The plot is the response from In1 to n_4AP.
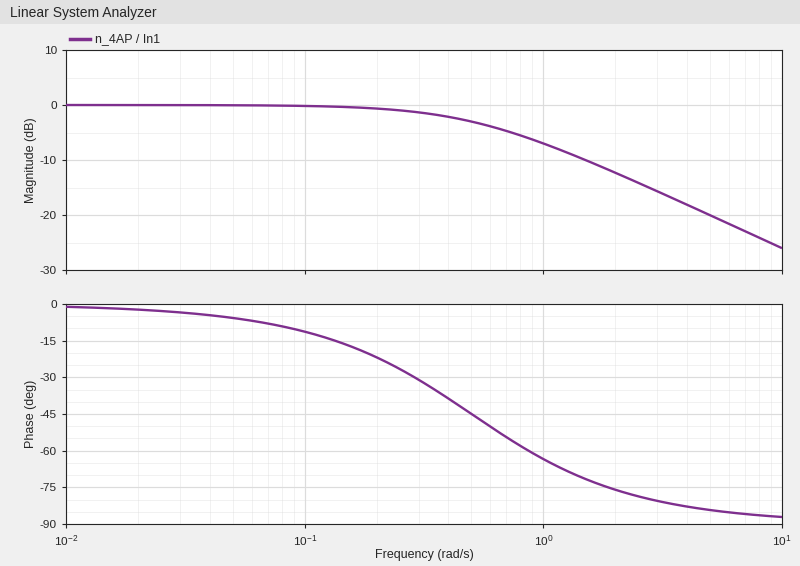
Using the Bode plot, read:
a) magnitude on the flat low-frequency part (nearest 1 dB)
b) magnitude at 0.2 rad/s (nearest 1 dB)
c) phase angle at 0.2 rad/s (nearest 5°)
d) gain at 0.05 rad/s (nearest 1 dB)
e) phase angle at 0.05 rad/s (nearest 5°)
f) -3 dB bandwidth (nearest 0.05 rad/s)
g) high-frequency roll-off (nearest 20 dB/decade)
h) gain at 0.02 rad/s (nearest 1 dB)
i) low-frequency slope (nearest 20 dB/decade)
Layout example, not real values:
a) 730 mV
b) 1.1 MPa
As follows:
a) 0 dB
b) -1 dB
c) -20°
d) 0 dB
e) -5°
f) 0.50 rad/s
g) -20 dB/decade
h) 0 dB
i) 0 dB/decade
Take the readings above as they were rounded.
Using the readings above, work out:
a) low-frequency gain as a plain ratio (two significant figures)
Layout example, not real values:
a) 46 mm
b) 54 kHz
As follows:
a) 1.0
